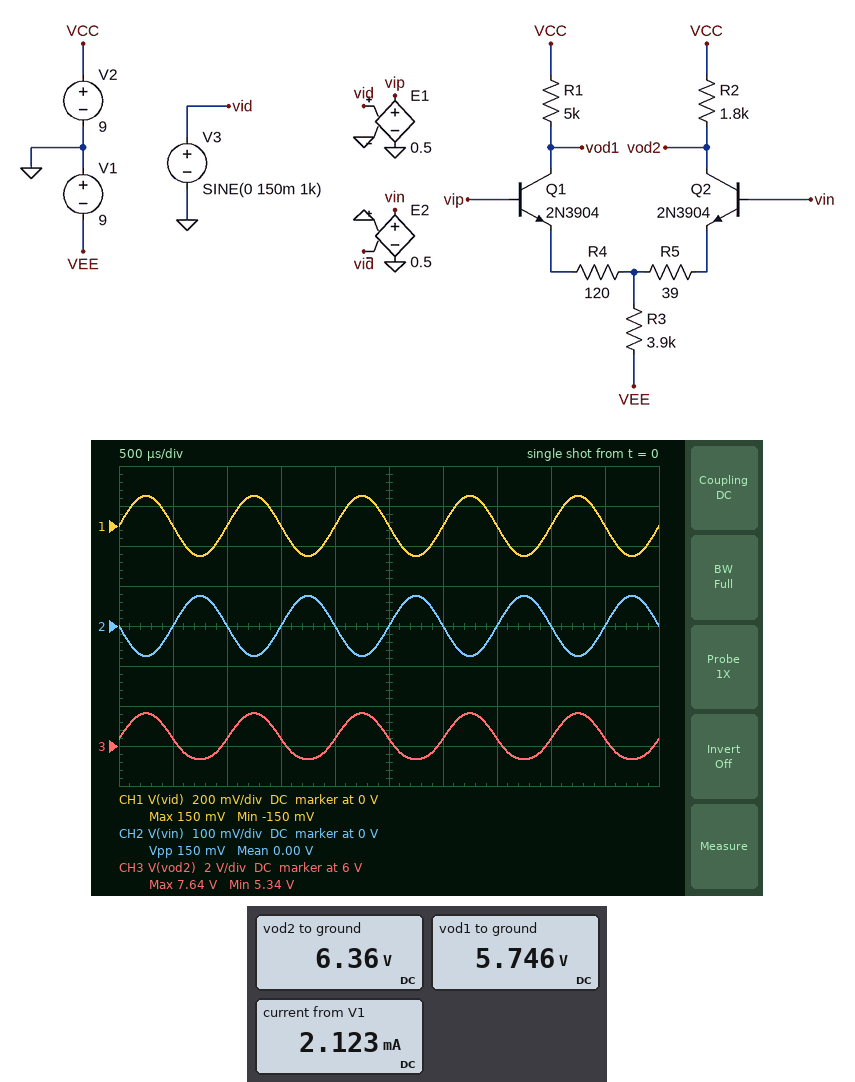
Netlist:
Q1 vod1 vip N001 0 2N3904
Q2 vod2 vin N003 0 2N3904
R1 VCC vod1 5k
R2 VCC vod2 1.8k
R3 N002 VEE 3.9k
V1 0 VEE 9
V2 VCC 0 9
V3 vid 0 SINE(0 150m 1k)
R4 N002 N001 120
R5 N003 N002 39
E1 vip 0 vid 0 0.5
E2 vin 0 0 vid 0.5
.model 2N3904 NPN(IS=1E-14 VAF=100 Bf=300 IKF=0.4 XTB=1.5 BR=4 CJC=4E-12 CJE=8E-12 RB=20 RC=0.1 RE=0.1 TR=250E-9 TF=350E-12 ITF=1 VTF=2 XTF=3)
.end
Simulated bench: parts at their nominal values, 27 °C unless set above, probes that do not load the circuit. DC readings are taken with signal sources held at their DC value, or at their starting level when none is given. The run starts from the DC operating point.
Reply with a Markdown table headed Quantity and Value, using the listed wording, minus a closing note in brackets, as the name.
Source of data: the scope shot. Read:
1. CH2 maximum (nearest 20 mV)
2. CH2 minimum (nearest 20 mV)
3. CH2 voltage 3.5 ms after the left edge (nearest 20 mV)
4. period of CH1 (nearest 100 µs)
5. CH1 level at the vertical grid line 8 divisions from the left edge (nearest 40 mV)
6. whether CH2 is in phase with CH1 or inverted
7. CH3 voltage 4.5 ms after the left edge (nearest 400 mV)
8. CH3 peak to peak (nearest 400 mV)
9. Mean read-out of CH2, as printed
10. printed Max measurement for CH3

| Quantity | Value |
|---|---|
| CH2 maximum | 80 mV |
| CH2 minimum | -80 mV |
| CH2 voltage 3.5 ms after the left edge | 0 V |
| period of CH1 | 1.0 ms |
| CH1 level at the vertical grid line 8 divisions from the left edge | 0 V |
| whether CH2 is in phase with CH1 or inverted | inverted |
| CH3 voltage 4.5 ms after the left edge | 6.4 V |
| CH3 peak to peak | 2.4 V |
| Mean read-out of CH2, as printed | 0.00 V |
| printed Max measurement for CH3 | 7.64 V |
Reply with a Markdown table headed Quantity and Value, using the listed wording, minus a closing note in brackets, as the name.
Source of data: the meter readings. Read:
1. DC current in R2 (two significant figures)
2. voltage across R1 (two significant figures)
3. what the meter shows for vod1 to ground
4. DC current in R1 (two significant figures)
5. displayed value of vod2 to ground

| Quantity | Value |
|---|---|
| DC current in R2 | 1.5 mA |
| voltage across R1 | 3.3 V |
| what the meter shows for vod1 to ground | 5.746 V |
| DC current in R1 | 650 µA |
| displayed value of vod2 to ground | 6.36 V |
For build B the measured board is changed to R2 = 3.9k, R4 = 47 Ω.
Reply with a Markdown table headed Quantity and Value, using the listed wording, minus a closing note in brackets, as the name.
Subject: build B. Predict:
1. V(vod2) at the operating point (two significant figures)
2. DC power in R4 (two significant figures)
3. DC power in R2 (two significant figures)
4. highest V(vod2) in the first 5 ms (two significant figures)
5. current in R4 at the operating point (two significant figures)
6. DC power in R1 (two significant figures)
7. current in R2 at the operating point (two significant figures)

| Quantity | Value |
|---|---|
| V(vod2) at the operating point | 4.6 V |
| DC power in R4 | 47 µW |
| DC power in R2 | 4.9 mW |
| highest V(vod2) in the first 5 ms | 8.3 V |
| current in R4 at the operating point | 1.0 mA |
| DC power in R1 | 5.0 mW |
| current in R2 at the operating point | 1.1 mA |
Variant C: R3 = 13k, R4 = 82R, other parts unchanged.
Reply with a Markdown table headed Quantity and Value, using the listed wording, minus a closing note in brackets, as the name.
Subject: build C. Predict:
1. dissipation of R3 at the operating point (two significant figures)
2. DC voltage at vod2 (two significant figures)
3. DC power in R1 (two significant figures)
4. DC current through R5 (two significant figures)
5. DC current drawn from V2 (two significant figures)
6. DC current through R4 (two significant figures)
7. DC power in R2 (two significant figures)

| Quantity | Value |
|---|---|
| dissipation of R3 at the operating point | 5.4 mW |
| DC voltage at vod2 | 8.3 V |
| DC power in R1 | 370 µW |
| DC current through R5 | 370 µA |
| DC current drawn from V2 | 640 µA |
| DC current through R4 | 270 µA |
| DC power in R2 | 250 µW |
